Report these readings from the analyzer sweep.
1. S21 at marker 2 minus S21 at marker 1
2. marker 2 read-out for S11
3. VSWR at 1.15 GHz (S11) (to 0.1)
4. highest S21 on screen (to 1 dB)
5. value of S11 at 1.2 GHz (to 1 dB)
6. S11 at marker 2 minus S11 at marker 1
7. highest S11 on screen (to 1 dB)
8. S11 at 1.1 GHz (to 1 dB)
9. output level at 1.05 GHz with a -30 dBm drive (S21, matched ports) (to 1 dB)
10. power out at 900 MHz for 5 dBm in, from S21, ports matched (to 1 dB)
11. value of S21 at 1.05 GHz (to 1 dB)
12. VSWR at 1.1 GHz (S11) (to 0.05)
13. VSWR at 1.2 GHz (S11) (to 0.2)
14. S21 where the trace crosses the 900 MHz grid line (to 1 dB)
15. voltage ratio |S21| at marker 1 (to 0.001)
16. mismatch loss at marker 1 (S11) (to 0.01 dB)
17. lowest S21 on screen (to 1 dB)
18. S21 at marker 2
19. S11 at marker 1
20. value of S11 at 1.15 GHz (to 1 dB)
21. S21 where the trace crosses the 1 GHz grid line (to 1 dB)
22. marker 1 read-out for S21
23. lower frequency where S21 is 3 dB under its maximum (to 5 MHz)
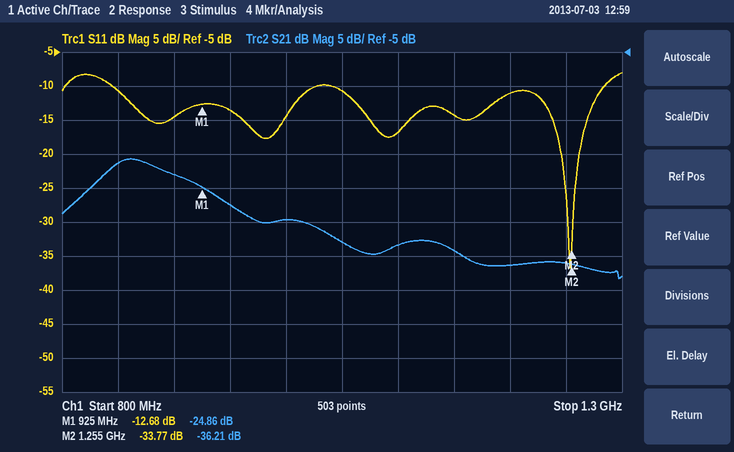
-11.35 dB
-33.77 dB
1.5
-21 dB
-11 dB
-21.09 dB
-8 dB
-17 dB
-63 dBm
-18 dBm
-33 dB
1.35
1.8
-23 dB
0.057
0.24 dB
-38 dB
-36.21 dB
-12.68 dB
-14 dB
-30 dB
-24.86 dB
835 MHz
